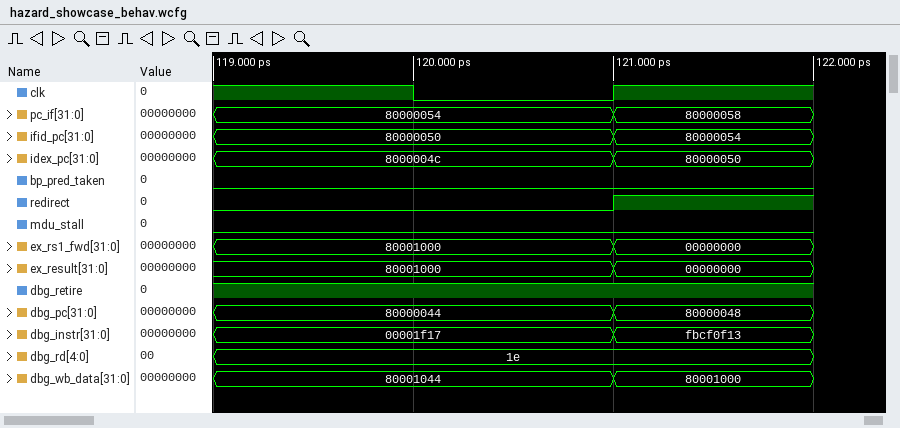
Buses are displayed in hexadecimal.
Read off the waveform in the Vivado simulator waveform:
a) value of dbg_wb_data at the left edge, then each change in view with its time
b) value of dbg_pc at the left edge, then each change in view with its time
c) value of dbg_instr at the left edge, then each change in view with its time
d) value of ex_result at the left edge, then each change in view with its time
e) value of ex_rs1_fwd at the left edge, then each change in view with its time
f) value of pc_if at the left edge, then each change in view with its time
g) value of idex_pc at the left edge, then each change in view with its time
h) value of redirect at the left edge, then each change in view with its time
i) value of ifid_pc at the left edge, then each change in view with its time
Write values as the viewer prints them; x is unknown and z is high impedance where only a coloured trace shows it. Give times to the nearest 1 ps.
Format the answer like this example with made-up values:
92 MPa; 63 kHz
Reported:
80001044, 80001000 at 121 ps; 80000044, 80000048 at 121 ps; 00001f17, fbcf0f13 at 121 ps; 80001000, 00000000 at 121 ps; 80001000, 00000000 at 121 ps; 80000054, 80000058 at 121 ps; 8000004c, 80000050 at 121 ps; 0, 1 at 121 ps; 80000050, 80000054 at 121 ps
